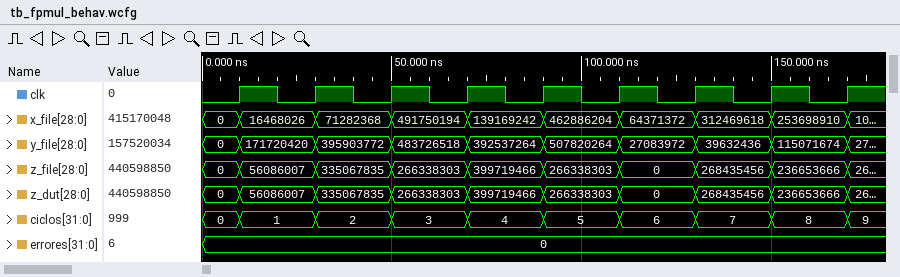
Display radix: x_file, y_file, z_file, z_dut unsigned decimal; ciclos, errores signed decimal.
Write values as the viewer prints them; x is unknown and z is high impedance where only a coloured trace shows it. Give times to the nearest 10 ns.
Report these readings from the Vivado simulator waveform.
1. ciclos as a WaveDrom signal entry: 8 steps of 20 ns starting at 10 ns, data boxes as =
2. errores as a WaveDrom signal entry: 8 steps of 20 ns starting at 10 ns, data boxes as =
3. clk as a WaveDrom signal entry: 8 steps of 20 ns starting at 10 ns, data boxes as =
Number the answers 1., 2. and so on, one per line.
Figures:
1. {name: 'ciclos', wave: '========', data: '1 2 3 4 5 6 7 8'}
2. {name: 'errores', wave: '=.......', data: '0'}
3. {name: 'clk', wave: 'p.......'}
